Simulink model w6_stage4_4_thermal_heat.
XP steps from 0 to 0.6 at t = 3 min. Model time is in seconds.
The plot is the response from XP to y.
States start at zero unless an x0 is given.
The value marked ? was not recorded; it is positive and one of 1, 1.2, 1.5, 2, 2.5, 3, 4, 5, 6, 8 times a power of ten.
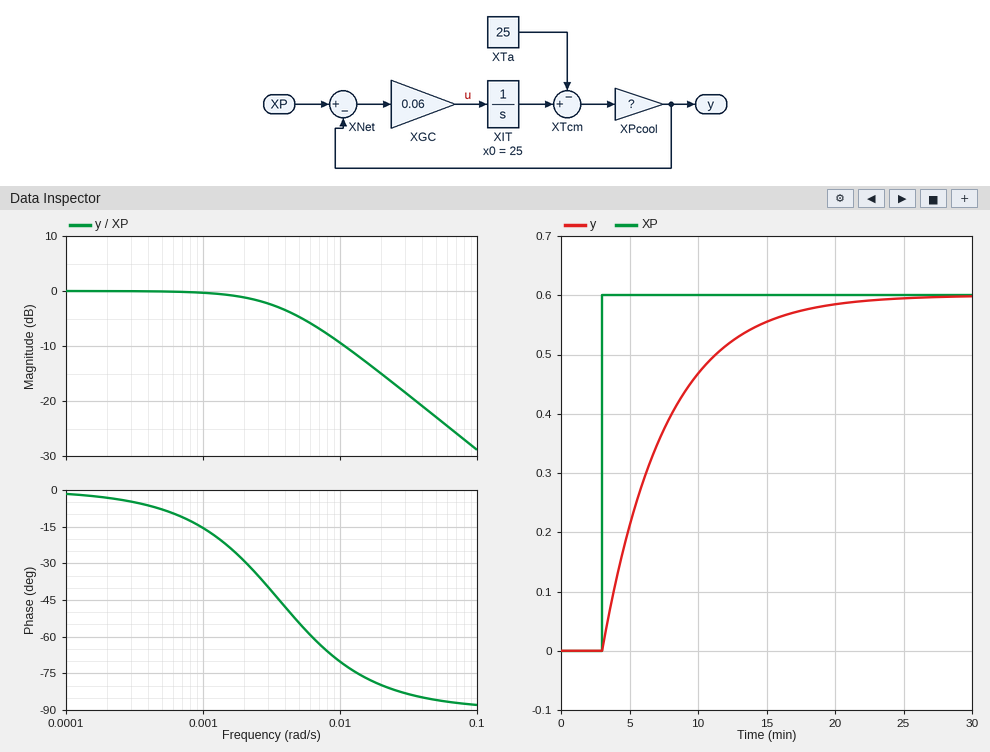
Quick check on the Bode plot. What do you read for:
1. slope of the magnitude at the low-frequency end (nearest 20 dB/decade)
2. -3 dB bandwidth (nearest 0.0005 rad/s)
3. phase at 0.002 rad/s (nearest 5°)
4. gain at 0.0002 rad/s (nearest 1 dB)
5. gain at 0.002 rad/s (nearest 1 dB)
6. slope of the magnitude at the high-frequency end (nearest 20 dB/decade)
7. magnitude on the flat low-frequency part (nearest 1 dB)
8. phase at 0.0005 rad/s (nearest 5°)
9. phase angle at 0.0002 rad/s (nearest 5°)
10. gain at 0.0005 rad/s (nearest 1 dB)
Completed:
0 dB/decade
0.0035 rad/s
-30°
0 dB
-1 dB
-20 dB/decade
0 dB
-10°
-5°
0 dB
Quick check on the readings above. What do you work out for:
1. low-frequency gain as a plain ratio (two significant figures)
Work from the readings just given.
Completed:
1.0
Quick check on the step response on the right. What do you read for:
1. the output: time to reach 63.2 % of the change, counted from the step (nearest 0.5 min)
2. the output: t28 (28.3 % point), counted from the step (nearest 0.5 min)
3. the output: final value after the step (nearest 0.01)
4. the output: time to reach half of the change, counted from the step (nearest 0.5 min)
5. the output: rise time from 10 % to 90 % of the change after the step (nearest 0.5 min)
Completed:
4.5 min
1.5 min
0.60
3.0 min
10.0 min
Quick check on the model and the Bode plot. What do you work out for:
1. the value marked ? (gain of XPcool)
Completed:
0.06
